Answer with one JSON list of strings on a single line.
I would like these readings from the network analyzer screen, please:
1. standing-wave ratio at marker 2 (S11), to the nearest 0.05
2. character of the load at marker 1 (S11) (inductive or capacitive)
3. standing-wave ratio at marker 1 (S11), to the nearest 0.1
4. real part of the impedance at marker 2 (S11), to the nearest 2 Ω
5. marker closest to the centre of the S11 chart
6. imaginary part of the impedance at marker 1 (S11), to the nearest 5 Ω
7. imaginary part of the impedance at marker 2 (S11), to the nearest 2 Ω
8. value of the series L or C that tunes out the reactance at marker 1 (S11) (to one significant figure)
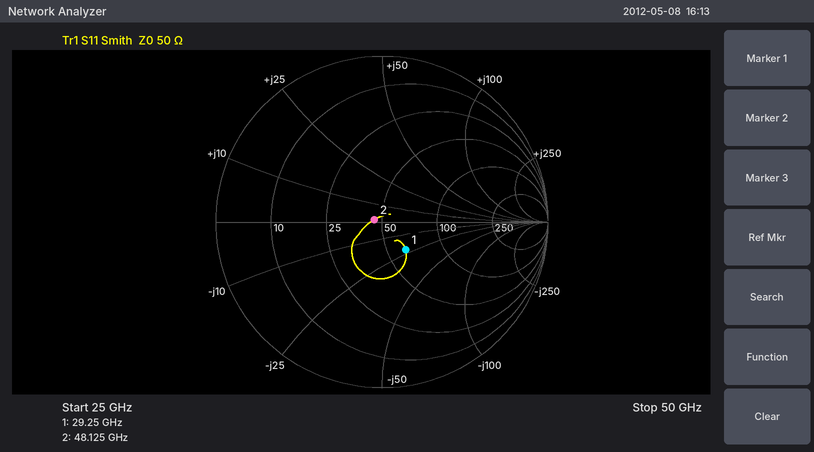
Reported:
["1.10", "capacitive", "1.6", "46 Ω", "marker 2", "-20 Ω", "+2 Ω", "100 pH"]
